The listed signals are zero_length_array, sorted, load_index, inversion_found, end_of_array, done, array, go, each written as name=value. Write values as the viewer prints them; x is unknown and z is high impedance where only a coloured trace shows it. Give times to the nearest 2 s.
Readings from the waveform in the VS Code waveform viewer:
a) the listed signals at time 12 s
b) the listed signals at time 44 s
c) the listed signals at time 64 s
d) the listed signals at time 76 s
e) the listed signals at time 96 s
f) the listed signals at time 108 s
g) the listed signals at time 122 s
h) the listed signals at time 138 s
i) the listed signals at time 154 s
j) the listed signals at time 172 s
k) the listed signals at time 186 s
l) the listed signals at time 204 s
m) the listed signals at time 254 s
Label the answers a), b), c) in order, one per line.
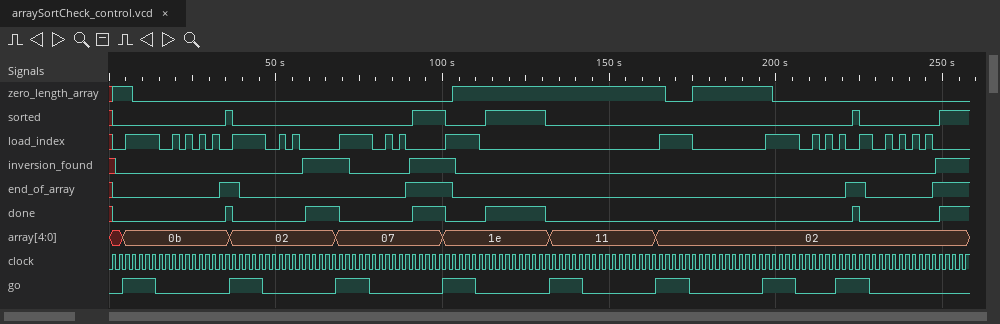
a) zero_length_array=0, sorted=0, load_index=1, inversion_found=0, end_of_array=0, done=0, array=0b, go=1
b) zero_length_array=0, sorted=0, load_index=1, inversion_found=0, end_of_array=0, done=0, array=02, go=1
c) zero_length_array=0, sorted=0, load_index=0, inversion_found=1, end_of_array=0, done=1, array=02, go=0
d) zero_length_array=0, sorted=0, load_index=1, inversion_found=0, end_of_array=0, done=0, array=07, go=1
e) zero_length_array=0, sorted=1, load_index=0, inversion_found=1, end_of_array=1, done=1, array=07, go=0
f) zero_length_array=1, sorted=0, load_index=1, inversion_found=0, end_of_array=0, done=0, array=1e, go=1
g) zero_length_array=1, sorted=1, load_index=0, inversion_found=0, end_of_array=0, done=1, array=1e, go=0
h) zero_length_array=1, sorted=0, load_index=0, inversion_found=0, end_of_array=0, done=0, array=11, go=1
i) zero_length_array=1, sorted=0, load_index=0, inversion_found=0, end_of_array=0, done=0, array=11, go=0
j) zero_length_array=0, sorted=0, load_index=1, inversion_found=0, end_of_array=0, done=0, array=02, go=1
k) zero_length_array=1, sorted=0, load_index=0, inversion_found=0, end_of_array=0, done=0, array=02, go=0
l) zero_length_array=0, sorted=0, load_index=1, inversion_found=0, end_of_array=0, done=0, array=02, go=1
m) zero_length_array=0, sorted=1, load_index=0, inversion_found=1, end_of_array=1, done=1, array=02, go=0
